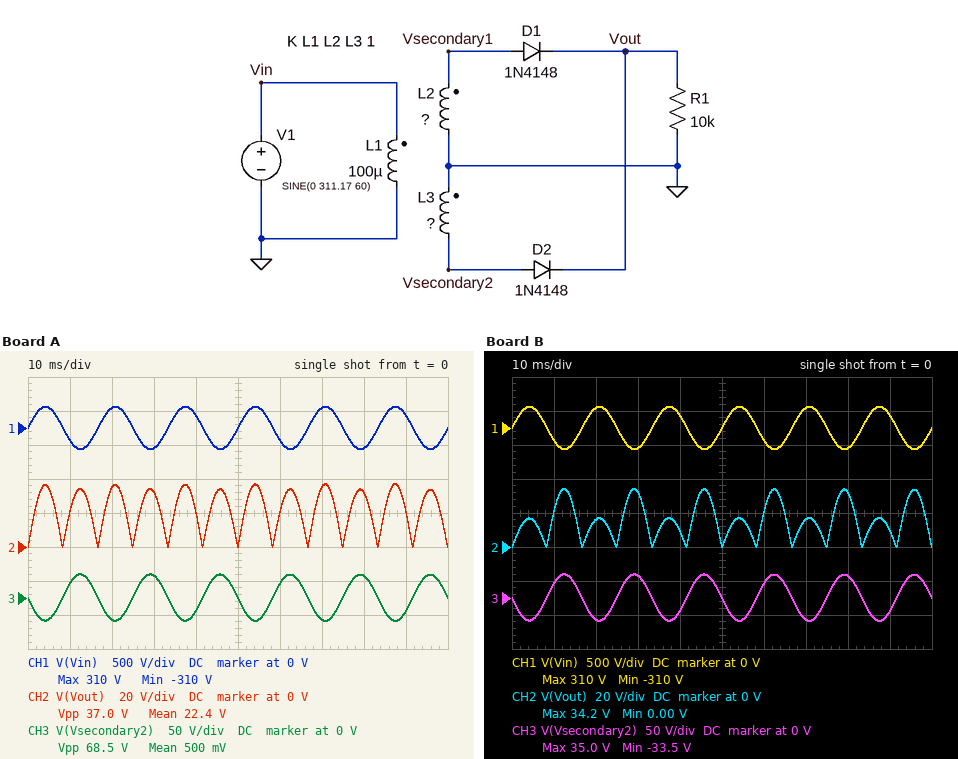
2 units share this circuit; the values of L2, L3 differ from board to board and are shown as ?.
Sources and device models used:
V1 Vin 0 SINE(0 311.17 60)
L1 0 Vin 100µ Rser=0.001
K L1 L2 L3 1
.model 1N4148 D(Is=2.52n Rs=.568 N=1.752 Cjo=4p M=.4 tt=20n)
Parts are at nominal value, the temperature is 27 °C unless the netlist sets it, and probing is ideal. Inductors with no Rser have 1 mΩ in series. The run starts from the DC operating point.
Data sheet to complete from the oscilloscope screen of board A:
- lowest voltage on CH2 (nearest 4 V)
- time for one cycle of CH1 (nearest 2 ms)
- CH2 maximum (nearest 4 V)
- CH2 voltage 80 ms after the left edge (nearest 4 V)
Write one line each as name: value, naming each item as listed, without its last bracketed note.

lowest voltage on CH2: 0 V
time for one cycle of CH1: 16 ms
CH2 maximum: 36 V
CH2 voltage 80 ms after the left edge: 32 V
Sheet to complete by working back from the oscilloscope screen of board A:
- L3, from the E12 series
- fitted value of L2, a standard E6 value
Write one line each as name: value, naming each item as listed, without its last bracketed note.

L3, from the E12 series: 1.2 µH
fitted value of L2, a standard E6 value: 1.5 µH
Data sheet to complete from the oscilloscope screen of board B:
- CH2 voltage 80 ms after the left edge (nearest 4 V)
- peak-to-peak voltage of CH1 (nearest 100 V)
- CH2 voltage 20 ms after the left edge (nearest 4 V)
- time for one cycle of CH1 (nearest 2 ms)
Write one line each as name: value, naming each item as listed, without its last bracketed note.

CH2 voltage 80 ms after the left edge: 32 V
peak-to-peak voltage of CH1: 600 V
CH2 voltage 20 ms after the left edge: 16 V
time for one cycle of CH1: 16 ms
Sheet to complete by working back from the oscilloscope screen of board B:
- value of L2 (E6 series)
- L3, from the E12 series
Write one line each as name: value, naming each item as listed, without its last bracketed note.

value of L2: 330 nH
L3, from the E12 series: 1.2 µH
